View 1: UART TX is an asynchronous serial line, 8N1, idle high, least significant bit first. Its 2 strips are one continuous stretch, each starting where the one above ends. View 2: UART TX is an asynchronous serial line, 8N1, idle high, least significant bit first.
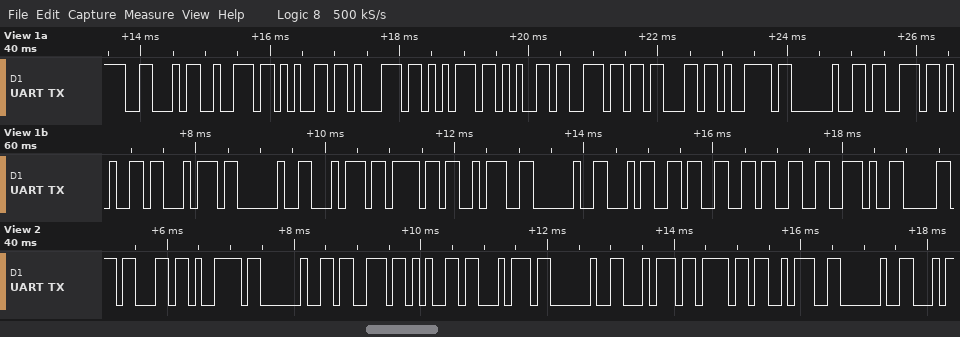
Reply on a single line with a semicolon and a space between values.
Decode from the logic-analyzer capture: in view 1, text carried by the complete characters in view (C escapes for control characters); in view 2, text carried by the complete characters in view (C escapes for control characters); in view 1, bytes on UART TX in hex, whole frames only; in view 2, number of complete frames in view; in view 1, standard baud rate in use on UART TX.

"Frequency set to: 433."; "cy set to: "; 0x46 0x72 0x65 0x71 0x75 0x65 0x6E 0x63 0x79 0x20 0x73 0x65 0x74 0x20 0x74 0x6F 0x3A 0x20 0x34 0x33 0x33 0x2E; 11; 9600 baud
